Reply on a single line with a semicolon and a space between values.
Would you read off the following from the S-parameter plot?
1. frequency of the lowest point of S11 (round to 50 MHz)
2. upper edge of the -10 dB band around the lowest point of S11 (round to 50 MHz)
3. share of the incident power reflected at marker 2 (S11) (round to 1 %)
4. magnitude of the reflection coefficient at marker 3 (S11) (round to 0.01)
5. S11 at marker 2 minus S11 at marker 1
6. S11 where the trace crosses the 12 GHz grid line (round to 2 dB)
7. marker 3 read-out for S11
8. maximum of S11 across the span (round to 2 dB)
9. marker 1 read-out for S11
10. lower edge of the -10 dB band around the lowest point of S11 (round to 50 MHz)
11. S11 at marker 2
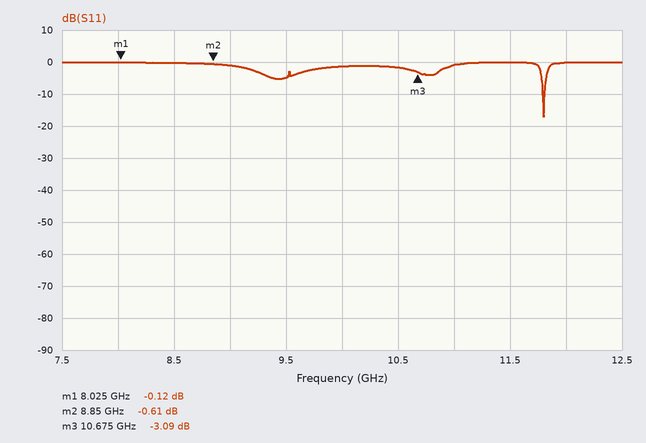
11.80 GHz; 11.80 GHz; 87 %; 0.70; -0.49 dB; 0 dB; -3.09 dB; 0 dB; -0.12 dB; 11.80 GHz; -0.61 dB
